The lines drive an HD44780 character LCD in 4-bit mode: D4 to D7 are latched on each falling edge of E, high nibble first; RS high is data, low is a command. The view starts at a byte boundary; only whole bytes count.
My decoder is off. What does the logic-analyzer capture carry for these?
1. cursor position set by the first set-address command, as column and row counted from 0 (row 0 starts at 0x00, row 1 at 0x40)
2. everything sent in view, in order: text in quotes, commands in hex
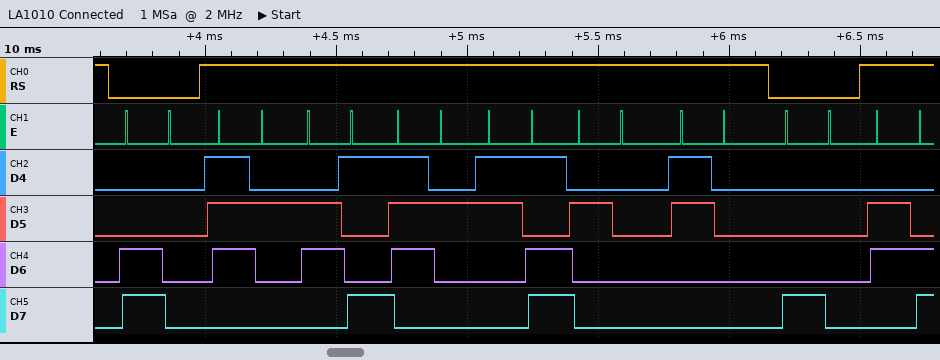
column 0, row 1
0xC0 "rir= 0" 0x80 "l"
